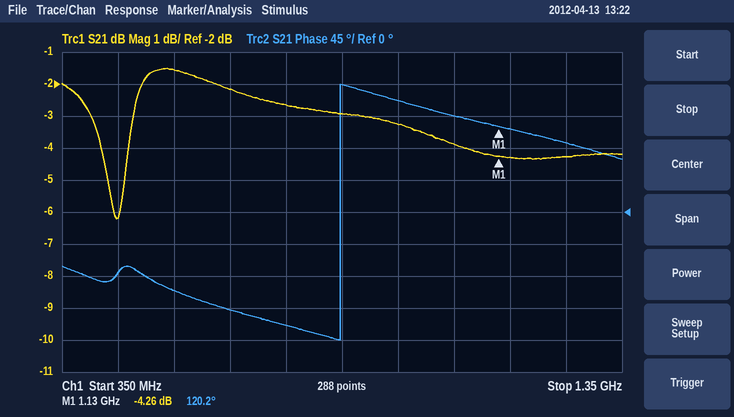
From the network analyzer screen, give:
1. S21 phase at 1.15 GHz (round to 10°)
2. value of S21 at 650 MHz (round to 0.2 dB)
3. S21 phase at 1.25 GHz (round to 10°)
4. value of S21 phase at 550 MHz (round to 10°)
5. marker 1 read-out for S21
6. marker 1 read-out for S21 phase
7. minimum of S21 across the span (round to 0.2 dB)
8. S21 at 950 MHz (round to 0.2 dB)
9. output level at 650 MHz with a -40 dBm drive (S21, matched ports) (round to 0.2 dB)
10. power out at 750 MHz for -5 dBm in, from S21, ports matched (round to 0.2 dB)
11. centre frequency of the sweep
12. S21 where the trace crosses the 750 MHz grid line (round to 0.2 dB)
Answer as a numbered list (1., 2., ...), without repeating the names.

1. 120°
2. -2.2 dB
3. 100°
4. -110°
5. -4.26 dB
6. 120.2°
7. -6.2 dB
8. -3.2 dB
9. -42.2 dBm
10. -7.6 dBm
11. 850 MHz
12. -2.6 dB
